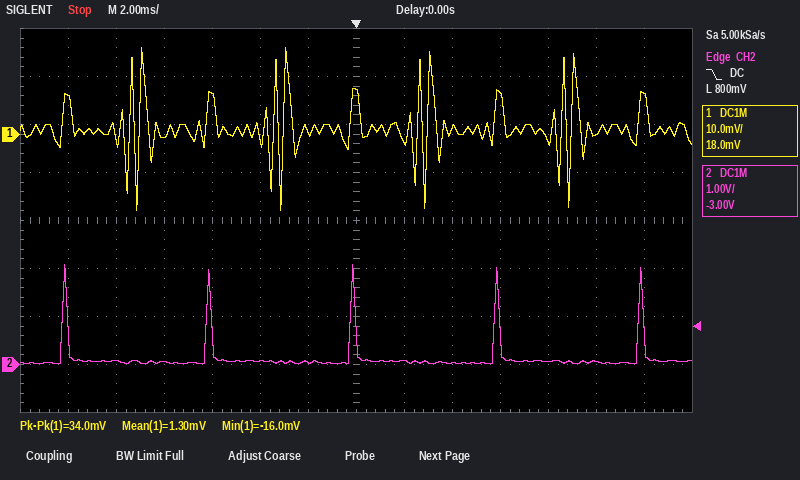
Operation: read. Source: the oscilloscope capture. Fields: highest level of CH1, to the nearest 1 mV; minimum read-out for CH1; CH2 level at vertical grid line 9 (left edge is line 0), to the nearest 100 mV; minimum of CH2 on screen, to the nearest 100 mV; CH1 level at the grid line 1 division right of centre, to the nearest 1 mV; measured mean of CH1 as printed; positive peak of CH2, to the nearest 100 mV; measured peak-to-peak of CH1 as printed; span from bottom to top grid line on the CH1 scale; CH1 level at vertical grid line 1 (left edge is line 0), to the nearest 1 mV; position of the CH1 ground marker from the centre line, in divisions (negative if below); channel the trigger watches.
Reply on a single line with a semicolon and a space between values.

18 mV; -16.0 mV; 0.0 V; 0.0 V; -2 mV; 1.30 mV; 2.1 V; 34.0 mV; 80 mV; 8 mV; +1.8 div; CH2
